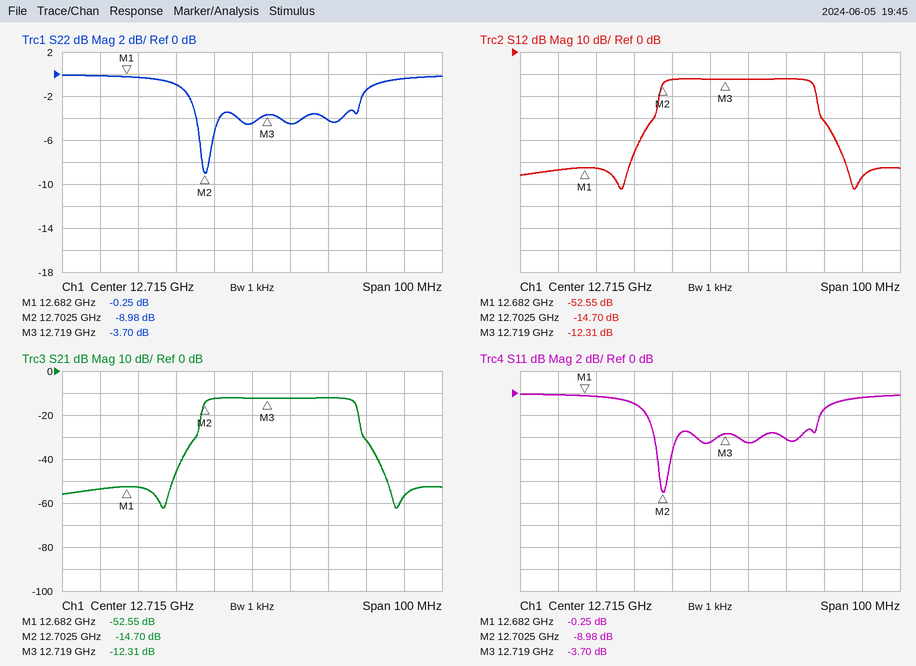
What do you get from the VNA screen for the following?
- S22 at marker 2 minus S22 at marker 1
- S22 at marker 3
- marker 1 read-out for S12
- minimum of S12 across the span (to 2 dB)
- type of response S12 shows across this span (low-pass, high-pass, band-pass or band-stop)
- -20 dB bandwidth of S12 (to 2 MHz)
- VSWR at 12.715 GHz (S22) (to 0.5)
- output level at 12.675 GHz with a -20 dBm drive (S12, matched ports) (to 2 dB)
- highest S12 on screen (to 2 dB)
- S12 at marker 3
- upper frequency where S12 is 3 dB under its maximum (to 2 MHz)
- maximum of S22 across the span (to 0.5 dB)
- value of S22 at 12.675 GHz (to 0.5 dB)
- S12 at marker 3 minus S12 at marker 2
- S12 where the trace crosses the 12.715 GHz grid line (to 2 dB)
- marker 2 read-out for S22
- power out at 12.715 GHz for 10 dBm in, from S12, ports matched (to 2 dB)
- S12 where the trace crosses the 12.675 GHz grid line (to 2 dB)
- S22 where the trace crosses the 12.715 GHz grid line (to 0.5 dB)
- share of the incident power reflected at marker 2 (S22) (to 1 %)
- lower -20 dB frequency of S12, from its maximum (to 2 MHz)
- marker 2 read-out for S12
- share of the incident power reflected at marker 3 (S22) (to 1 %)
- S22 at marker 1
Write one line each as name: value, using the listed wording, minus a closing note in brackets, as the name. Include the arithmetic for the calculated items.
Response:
S22 at marker 2 minus S22 at marker 1: -8.98 − (-0.25) = -8.73 dB
S22 at marker 3: -3.70 dB
marker 1 read-out for S12: -52.55 dB
minimum of S12 across the span: -62 dB
type of response S12 shows across this span: band-pass
-20 dB bandwidth of S12: 12.746 GHz − 12.700 GHz = 46 MHz
VSWR at 12.715 GHz (S22): |Γ| = 10^(-4.5/20) = 0.5957; VSWR = (1 + 0.5957)/(1 − 0.5957) ≈ 4.0
output level at 12.675 GHz with a -20 dBm drive (S12, matched ports): -20 dBm + (-54 dB) = -74 dBm
highest S12 on screen: -12 dB
S12 at marker 3: -12.31 dB
upper frequency where S12 is 3 dB under its maximum: 12.742 GHz
maximum of S22 across the span: 0.0 dB
value of S22 at 12.675 GHz: 0.0 dB
S12 at marker 3 minus S12 at marker 2: -12.31 − (-14.7) = 2.39 dB
S12 where the trace crosses the 12.715 GHz grid line: -12 dB
marker 2 read-out for S22: -8.98 dB
power out at 12.715 GHz for 10 dBm in, from S12, ports matched: 10 dBm + (-12 dB) = -2 dBm
S12 where the trace crosses the 12.675 GHz grid line: -54 dB
S22 where the trace crosses the 12.715 GHz grid line: -4.5 dB
share of the incident power reflected at marker 2 (S22): 10^(-8.98/10) ≈ 13 %
lower -20 dB frequency of S12, from its maximum: 12.700 GHz
marker 2 read-out for S12: -14.70 dB
share of the incident power reflected at marker 3 (S22): 10^(-3.7/10) ≈ 43 %
S22 at marker 1: -0.25 dB
